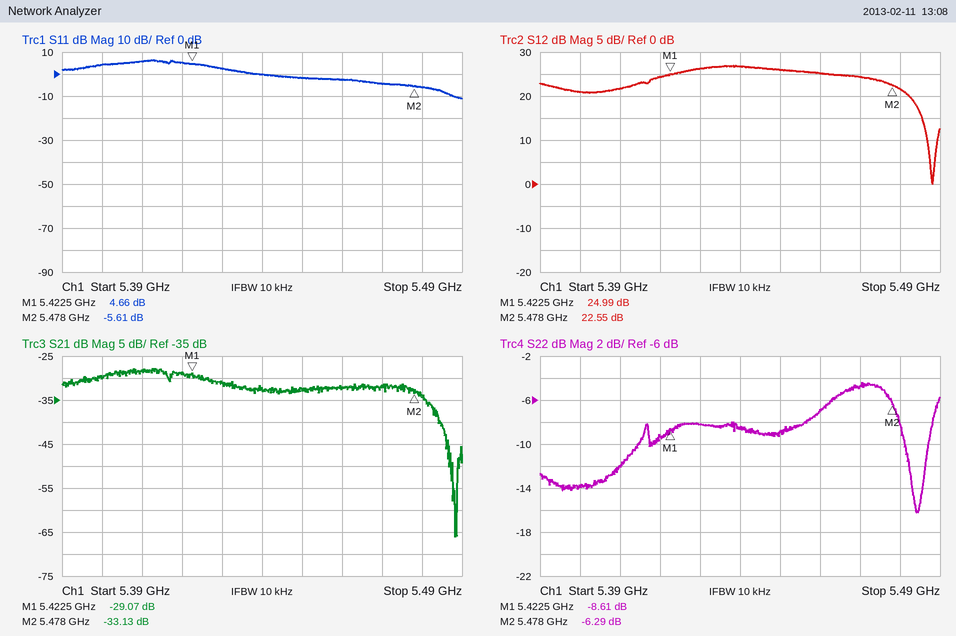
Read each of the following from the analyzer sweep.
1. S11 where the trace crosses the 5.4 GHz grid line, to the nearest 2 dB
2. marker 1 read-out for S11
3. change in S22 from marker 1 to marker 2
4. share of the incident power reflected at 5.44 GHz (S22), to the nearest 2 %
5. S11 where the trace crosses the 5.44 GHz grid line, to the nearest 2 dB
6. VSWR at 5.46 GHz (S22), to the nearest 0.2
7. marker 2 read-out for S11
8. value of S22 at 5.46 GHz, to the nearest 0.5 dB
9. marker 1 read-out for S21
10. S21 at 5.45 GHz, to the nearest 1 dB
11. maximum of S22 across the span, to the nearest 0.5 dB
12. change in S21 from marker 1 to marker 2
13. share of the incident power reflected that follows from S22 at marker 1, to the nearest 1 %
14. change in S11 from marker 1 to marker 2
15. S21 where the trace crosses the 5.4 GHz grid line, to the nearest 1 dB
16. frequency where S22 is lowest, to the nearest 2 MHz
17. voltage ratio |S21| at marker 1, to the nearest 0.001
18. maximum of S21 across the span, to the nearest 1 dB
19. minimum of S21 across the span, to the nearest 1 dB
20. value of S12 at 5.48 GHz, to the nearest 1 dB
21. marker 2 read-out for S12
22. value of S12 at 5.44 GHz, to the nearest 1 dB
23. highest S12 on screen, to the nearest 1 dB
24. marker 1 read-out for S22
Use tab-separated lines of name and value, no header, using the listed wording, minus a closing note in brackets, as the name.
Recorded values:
S11 where the trace crosses the 5.4 GHz grid line, to the nearest 2 dB	4 dB
marker 1 read-out for S11	4.66 dB
change in S22 from marker 1 to marker 2	2.32 dB
share of the incident power reflected at 5.44 GHz (S22), to the nearest 2 %	14 %
S11 where the trace crosses the 5.44 GHz grid line, to the nearest 2 dB	0 dB
VSWR at 5.46 GHz (S22), to the nearest 0.2	2.6
marker 2 read-out for S11	-5.61 dB
value of S22 at 5.46 GHz, to the nearest 0.5 dB	-7.0 dB
marker 1 read-out for S21	-29.07 dB
S21 at 5.45 GHz, to the nearest 1 dB	-33 dB
maximum of S22 across the span, to the nearest 0.5 dB	-4.5 dB
change in S21 from marker 1 to marker 2	-4.06 dB
share of the incident power reflected that follows from S22 at marker 1, to the nearest 1 %	14 %
change in S11 from marker 1 to marker 2	-10.27 dB
S21 where the trace crosses the 5.4 GHz grid line, to the nearest 1 dB	-30 dB
frequency where S22 is lowest, to the nearest 2 MHz	5.484 GHz
voltage ratio |S21| at marker 1, to the nearest 0.001	0.035
maximum of S21 across the span, to the nearest 1 dB	-28 dB
minimum of S21 across the span, to the nearest 1 dB	-66 dB
value of S12 at 5.48 GHz, to the nearest 1 dB	22 dB
marker 2 read-out for S12	22.55 dB
value of S12 at 5.44 GHz, to the nearest 1 dB	27 dB
highest S12 on screen, to the nearest 1 dB	27 dB
marker 1 read-out for S22	-8.61 dB
